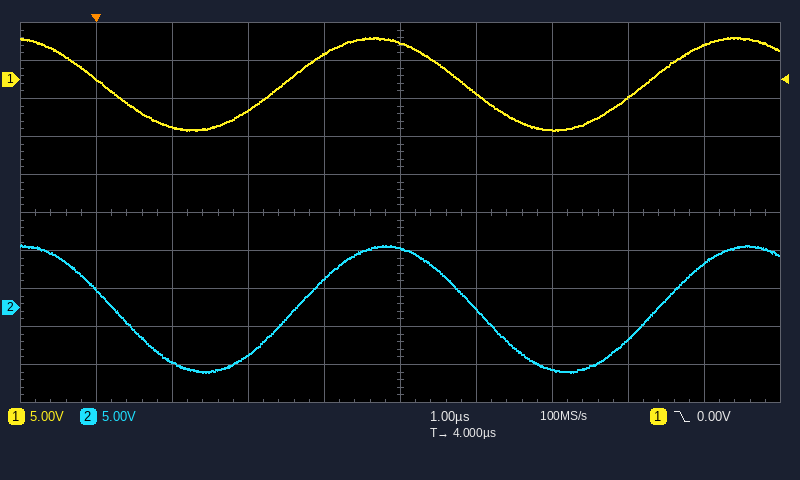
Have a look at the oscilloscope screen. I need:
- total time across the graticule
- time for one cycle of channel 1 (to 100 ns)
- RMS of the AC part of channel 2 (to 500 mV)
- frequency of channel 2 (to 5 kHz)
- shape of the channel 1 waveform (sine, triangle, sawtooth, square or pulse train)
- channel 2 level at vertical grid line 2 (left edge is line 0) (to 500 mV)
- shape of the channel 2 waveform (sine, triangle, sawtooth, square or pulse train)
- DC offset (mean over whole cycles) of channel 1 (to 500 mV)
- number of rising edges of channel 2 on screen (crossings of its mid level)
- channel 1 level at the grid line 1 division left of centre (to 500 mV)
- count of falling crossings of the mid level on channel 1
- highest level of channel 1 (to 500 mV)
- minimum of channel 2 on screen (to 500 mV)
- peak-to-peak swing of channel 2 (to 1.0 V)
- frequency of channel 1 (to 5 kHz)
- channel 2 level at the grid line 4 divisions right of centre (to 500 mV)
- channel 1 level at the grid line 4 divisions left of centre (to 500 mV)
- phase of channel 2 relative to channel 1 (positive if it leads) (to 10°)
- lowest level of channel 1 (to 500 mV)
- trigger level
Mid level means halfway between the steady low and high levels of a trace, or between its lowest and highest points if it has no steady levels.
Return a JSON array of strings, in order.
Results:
["10 µs", "4.8 µs", "6.0 V", "210 kHz", "sine", "-7.0 V", "sine", "-500 mV", "2", "3.5 V", "2", "5.5 V", "-8.5 V", "17.0 V", "210 kHz", "6.0 V", "0.0 V", "-10°", "-6.5 V", "0.00 V"]
